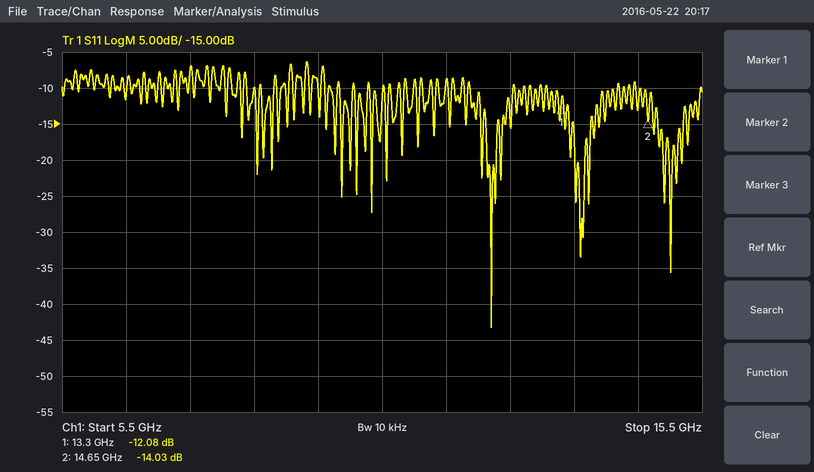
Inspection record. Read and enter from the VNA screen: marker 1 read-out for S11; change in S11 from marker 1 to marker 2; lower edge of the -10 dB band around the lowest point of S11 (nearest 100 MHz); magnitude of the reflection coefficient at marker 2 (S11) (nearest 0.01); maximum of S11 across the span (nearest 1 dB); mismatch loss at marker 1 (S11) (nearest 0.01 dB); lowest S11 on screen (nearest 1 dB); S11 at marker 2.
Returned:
-12.08 dB
-1.95 dB
11.9 GHz
0.20
-6 dB
0.28 dB
-43 dB
-14.03 dB
